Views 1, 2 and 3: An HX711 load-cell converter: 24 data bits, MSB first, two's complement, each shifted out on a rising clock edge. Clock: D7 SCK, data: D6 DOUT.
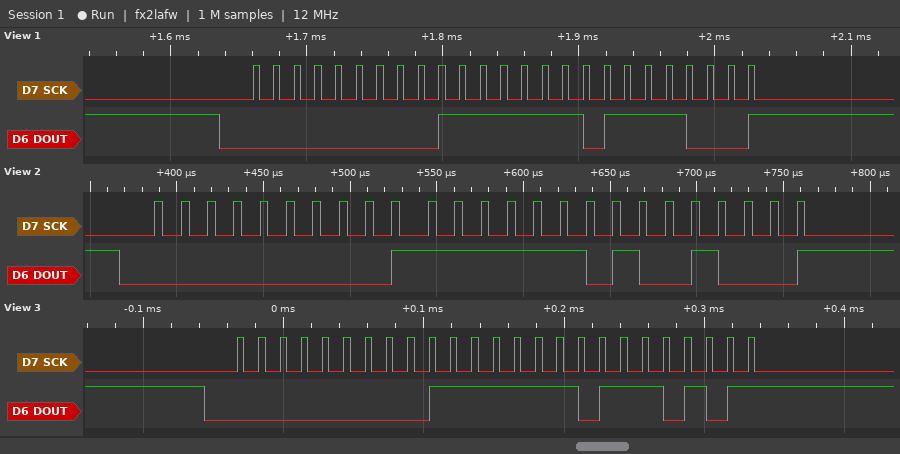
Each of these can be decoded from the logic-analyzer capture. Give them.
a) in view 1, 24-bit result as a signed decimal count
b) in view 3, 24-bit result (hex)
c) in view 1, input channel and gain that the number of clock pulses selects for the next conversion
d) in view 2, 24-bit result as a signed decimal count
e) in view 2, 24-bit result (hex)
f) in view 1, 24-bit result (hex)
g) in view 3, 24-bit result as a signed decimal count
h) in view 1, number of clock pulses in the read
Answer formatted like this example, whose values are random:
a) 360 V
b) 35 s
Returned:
a) 32632
b) 0x007F75
c) channel A, gain 128
d) 32584
e) 0x007F48
f) 0x007F78
g) 32629
h) 25
